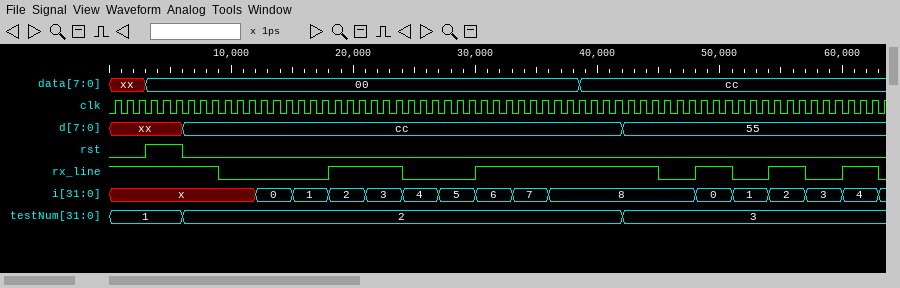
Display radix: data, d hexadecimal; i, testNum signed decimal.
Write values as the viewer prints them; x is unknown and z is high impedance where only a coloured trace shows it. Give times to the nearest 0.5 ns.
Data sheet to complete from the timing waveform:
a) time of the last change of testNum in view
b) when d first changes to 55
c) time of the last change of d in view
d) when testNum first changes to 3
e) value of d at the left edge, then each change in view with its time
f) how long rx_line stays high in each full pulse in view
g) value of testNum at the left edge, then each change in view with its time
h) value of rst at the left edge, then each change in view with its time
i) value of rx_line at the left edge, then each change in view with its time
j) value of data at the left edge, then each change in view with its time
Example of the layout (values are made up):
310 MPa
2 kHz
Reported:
42 ns
42 ns
42 ns
42 ns
xx, cc at 6 ns, 55 at 42 ns
6 ns, 15 ns, 3 ns, 3 ns, 3 ns
1, 2 at 6 ns, 3 at 42 ns
0, 1 at 3 ns, 0 at 6 ns
1, 0 at 9 ns, 1 at 18 ns, 0 at 24 ns, 1 at 30 ns, 0 at 45 ns, 1 at 48 ns, 0 at 51 ns, 1 at 54 ns, 0 at 57 ns, 1 at 60 ns, 0 at 63 ns
xx, 00 at 3 ns, cc at 38.5 ns
